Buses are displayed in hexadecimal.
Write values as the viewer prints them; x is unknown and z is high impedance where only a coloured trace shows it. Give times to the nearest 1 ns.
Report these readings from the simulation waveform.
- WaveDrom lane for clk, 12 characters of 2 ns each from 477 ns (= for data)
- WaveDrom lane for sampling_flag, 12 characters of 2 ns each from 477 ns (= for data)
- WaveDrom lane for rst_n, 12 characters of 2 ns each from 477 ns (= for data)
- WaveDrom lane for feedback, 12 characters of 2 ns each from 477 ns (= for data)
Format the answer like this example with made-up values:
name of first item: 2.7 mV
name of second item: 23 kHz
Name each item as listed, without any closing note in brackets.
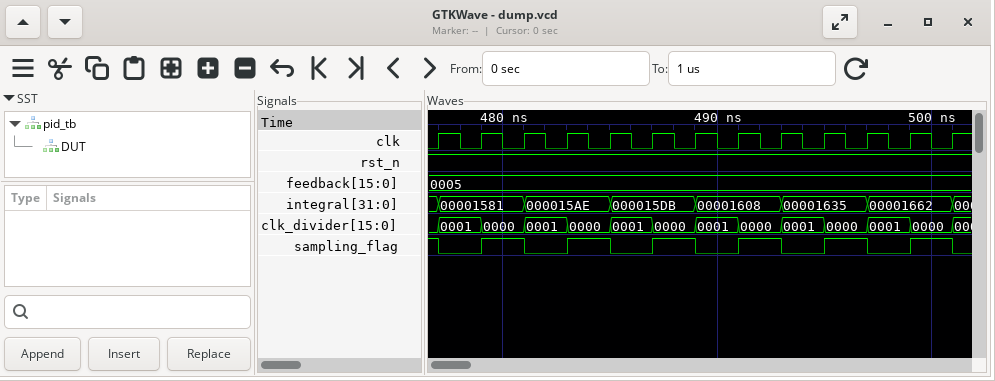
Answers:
WaveDrom lane for clk, 12 characters of 2 ns each from 477 ns: {name: 'clk', wave: 'p...........'}
WaveDrom lane for sampling_flag, 12 characters of 2 ns each from 477 ns: {name: 'sampling_flag', wave: '010101010101'}
WaveDrom lane for rst_n, 12 characters of 2 ns each from 477 ns: {name: 'rst_n', wave: '1...........'}
WaveDrom lane for feedback, 12 characters of 2 ns each from 477 ns: {name: 'feedback', wave: '=...........', data: '0005'}
